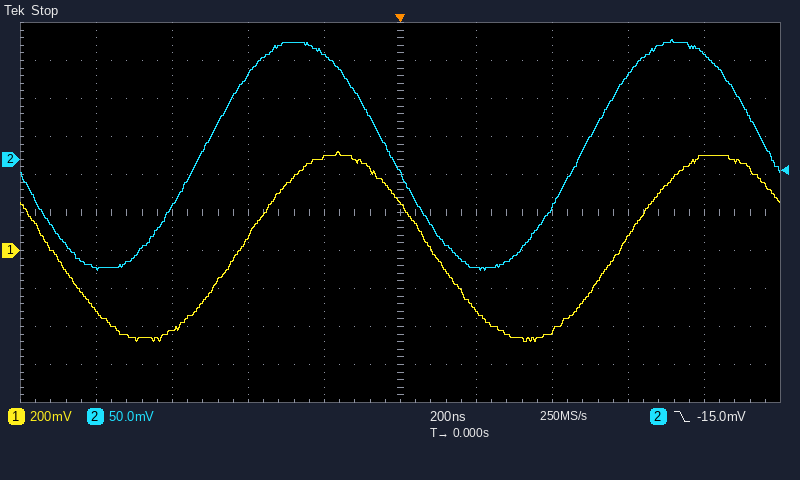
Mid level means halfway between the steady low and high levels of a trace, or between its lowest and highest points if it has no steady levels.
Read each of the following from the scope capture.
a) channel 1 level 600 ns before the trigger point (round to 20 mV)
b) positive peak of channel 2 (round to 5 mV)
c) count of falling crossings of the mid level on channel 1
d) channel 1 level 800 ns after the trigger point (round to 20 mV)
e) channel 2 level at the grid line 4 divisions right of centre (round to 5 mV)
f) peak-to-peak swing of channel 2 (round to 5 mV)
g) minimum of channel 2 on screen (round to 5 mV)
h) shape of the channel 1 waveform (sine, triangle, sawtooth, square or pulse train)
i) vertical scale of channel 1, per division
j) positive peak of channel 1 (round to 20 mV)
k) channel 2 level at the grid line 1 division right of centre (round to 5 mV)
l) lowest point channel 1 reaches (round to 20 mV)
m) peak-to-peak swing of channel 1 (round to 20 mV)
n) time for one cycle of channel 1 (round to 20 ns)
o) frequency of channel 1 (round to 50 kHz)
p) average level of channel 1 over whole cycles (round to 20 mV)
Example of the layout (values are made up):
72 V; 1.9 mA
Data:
-420 mV; 160 mV; 2; 500 mV; 140 mV; 305 mV; -145 mV; sine; 200 mV; 520 mV; -145 mV; -480 mV; 1.00 V; 1.00 µs; 1.00 MHz; 20 mV
